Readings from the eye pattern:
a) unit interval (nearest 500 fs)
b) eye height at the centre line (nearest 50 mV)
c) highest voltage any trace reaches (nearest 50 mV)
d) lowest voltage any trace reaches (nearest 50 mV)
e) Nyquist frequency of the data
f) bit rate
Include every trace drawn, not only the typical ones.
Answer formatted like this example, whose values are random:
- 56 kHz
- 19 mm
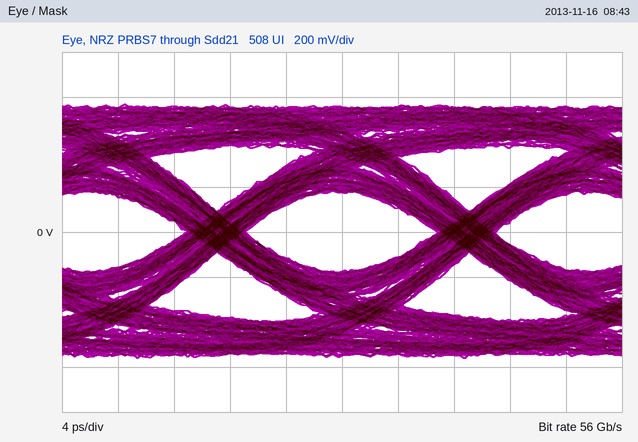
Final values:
- 18.0 ps
- 350 mV
- 550 mV
- -550 mV
- 28 GHz
- 56 Gb/s
